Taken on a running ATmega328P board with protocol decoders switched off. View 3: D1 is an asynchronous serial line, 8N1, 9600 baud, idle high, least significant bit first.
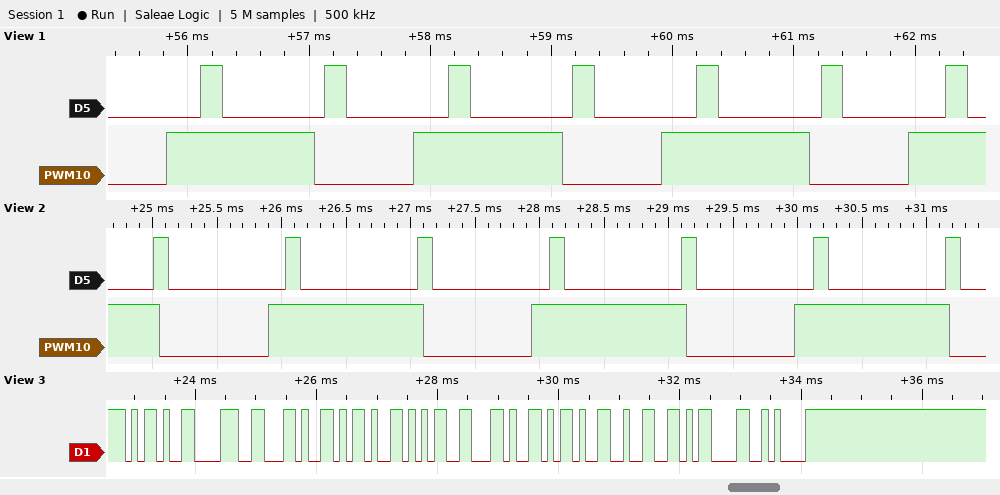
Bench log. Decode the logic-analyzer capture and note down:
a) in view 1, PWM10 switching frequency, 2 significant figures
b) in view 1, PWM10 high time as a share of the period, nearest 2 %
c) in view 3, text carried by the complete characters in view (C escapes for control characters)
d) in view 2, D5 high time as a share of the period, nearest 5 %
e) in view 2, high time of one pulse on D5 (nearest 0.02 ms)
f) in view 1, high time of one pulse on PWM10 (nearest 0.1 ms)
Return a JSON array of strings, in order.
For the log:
["490 Hz", "60 %", "\"-8,-5,-2\\r\\n\"", "10 %", "0.12 ms", "1.2 ms"]
